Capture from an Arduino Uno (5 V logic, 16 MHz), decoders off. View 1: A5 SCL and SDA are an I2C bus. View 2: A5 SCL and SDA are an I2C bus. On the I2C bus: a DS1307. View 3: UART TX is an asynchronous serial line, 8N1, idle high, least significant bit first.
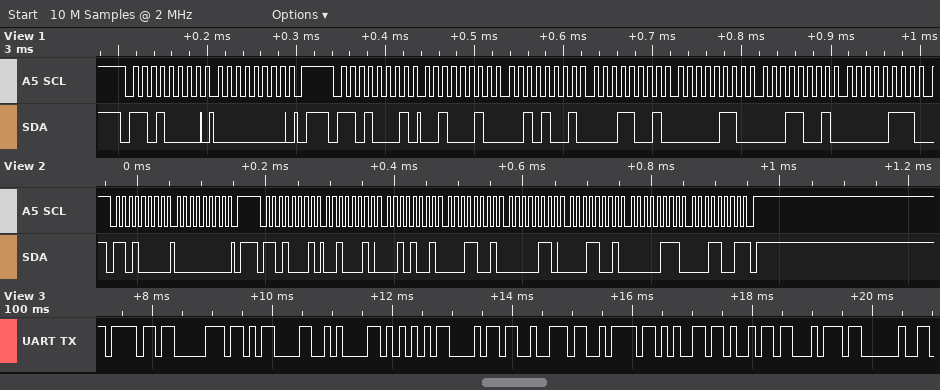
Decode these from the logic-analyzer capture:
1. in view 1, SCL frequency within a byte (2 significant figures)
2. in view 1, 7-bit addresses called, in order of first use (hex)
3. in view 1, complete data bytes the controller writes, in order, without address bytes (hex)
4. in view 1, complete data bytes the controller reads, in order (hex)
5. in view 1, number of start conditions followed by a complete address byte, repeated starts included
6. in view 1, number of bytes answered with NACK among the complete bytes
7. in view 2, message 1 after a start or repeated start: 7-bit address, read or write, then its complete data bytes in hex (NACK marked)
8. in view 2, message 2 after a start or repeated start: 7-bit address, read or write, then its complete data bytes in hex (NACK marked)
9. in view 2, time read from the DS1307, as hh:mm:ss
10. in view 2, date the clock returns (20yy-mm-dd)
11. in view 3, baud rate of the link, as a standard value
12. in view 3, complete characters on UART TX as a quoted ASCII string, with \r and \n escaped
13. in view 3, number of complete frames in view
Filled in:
100 kHz
0x68
00
22 29 19 06 19 07
2
0
0x68 write: 00
0x68 read: 22 29 19 06 19 07 19 NACK
19:29:22
2019-07-19
9600 baud
"op\r\nUhrzeit "
12
